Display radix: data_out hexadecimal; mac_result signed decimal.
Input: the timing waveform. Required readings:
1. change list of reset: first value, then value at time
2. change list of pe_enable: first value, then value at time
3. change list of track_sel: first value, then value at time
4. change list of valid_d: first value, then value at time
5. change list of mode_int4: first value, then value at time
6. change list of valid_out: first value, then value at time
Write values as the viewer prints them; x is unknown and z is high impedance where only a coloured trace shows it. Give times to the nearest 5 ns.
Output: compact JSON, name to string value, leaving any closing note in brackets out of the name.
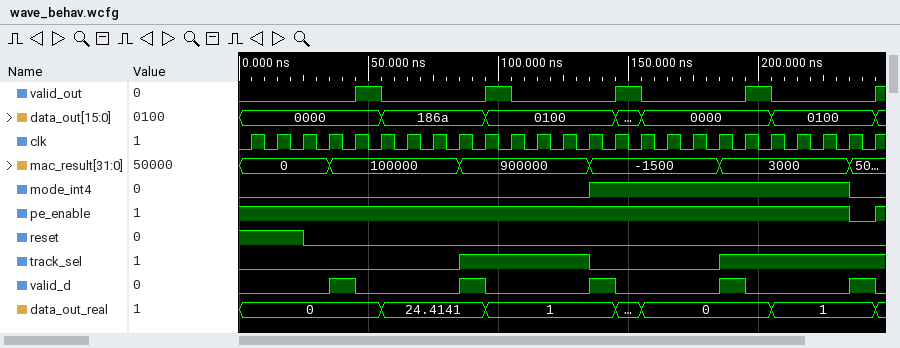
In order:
{"change list of reset: first value, then value at time": "1, 0 at 25 ns", "change list of pe_enable: first value, then value at time": "1, 0 at 235 ns, 1 at 245 ns", "change list of track_sel: first value, then value at time": "0, 1 at 85 ns, 0 at 135 ns, 1 at 185 ns", "change list of valid_d: first value, then value at time": "0, 1 at 35 ns, 0 at 45 ns, 1 at 85 ns, 0 at 95 ns, 1 at 135 ns, 0 at 145 ns, 1 at 185 ns, 0 at 195 ns, 1 at 235 ns, 0 at 245 ns", "change list of mode_int4: first value, then value at time": "0, 1 at 135 ns, 0 at 235 ns", "change list of valid_out: first value, then value at time": "0, 1 at 45 ns, 0 at 55 ns, 1 at 95 ns, 0 at 105 ns, 1 at 145 ns, 0 at 155 ns, 1 at 195 ns, 0 at 205 ns, 1 at 245 ns"}
